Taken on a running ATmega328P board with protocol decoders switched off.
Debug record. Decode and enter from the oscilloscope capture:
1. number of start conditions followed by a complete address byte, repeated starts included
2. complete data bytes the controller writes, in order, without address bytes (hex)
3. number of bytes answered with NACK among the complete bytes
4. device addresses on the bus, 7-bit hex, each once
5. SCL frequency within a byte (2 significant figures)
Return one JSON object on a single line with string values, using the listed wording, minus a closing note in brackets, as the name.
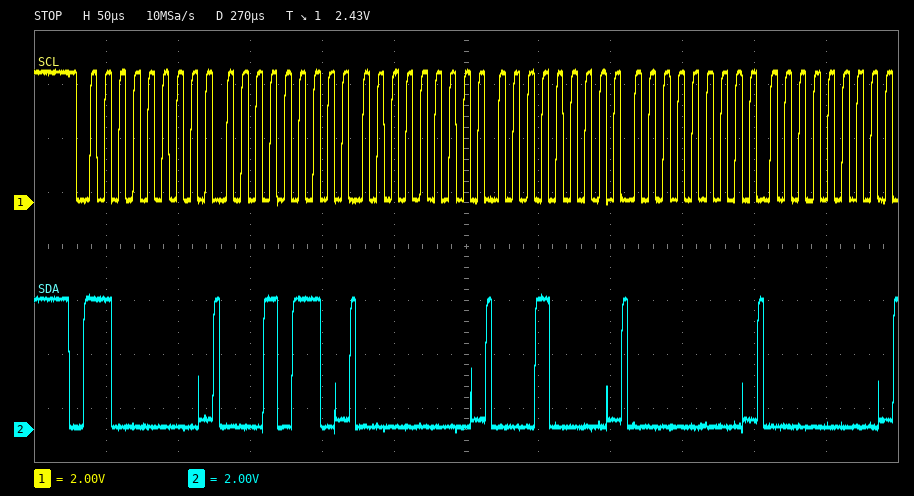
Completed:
{"number of start conditions followed by a complete address byte, repeated starts included": "1", "complete data bytes the controller writes, in order, without address bytes": "16 00 10 00 00", "number of bytes answered with NACK among the complete bytes": "0", "device addresses on the bus, 7-bit hex, each once": "0x60", "SCL frequency within a byte": "100 kHz"}
